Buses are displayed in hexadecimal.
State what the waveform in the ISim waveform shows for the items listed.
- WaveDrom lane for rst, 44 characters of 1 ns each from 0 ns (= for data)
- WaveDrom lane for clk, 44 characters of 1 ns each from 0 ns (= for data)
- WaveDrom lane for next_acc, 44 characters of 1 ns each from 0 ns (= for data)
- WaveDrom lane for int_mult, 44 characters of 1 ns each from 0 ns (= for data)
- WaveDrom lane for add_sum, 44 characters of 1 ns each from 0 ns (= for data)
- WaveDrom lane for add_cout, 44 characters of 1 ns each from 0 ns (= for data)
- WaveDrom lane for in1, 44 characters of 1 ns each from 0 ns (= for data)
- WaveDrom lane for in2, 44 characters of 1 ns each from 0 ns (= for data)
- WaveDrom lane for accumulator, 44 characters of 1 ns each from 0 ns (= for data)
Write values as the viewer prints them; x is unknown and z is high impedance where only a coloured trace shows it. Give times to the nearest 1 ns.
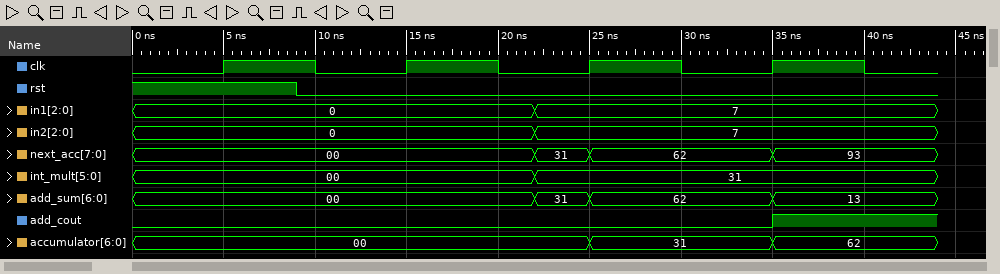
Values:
{name: 'rst', wave: '1........0..................................'}
{name: 'clk', wave: '0....1....0....1....0....1....0....1....0...'}
{name: 'next_acc', wave: '=.....................=..=.........=........', data: '00 31 62 93'}
{name: 'int_mult', wave: '=.....................=.....................', data: '00 31'}
{name: 'add_sum', wave: '=.....................=..=.........=........', data: '00 31 62 13'}
{name: 'add_cout', wave: '0..................................1........'}
{name: 'in1', wave: '=.....................=.....................', data: '0 7'}
{name: 'in2', wave: '=.....................=.....................', data: '0 7'}
{name: 'accumulator', wave: '=........................=.........=........', data: '00 31 62'}
